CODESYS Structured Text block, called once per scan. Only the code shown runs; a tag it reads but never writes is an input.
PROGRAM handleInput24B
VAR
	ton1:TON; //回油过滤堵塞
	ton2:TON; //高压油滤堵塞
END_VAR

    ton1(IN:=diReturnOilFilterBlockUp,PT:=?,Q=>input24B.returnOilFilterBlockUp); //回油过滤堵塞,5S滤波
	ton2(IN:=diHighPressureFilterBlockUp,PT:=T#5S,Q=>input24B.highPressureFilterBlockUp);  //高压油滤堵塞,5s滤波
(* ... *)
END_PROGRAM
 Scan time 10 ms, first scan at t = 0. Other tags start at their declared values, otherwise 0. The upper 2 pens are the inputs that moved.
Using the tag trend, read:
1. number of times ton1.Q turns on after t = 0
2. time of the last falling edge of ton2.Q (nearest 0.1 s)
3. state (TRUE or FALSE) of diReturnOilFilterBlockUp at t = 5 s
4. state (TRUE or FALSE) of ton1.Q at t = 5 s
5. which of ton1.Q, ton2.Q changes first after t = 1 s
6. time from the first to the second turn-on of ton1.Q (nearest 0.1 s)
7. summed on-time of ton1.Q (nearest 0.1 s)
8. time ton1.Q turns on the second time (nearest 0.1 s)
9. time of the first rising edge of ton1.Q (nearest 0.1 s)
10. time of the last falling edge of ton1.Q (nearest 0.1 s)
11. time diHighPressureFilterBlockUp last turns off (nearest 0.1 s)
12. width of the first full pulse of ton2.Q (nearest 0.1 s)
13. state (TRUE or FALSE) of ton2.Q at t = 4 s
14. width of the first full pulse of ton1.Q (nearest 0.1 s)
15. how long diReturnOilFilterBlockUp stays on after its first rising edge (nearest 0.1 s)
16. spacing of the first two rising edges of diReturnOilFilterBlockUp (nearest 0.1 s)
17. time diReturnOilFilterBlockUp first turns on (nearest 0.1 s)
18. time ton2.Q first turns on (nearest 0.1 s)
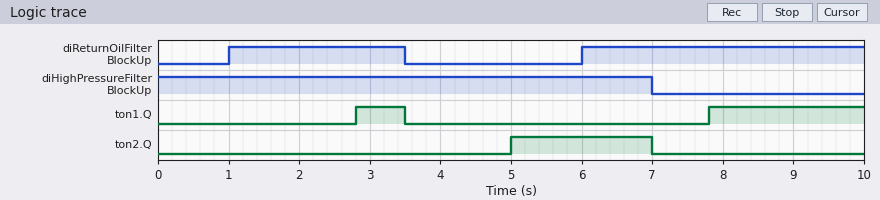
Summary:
2
7.0 s
FALSE
FALSE
ton1.Q
5.0 s
2.9 s
7.8 s
2.8 s
3.5 s
7.0 s
2.0 s
FALSE
0.7 s
2.5 s
5.0 s
1.0 s
5.0 s
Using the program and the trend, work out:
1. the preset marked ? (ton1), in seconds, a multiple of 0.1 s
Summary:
1.8 s
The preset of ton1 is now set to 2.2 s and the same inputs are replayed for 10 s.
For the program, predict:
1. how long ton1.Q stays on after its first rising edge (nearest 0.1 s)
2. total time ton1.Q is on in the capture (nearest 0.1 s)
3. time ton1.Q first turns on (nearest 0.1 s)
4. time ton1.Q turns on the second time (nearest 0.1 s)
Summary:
0.3 s
2.1 s
3.2 s
8.2 s
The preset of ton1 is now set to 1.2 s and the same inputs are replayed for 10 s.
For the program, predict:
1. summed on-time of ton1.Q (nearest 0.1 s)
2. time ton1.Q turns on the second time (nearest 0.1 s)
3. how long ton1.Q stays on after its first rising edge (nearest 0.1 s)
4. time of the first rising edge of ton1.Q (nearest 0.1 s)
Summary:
4.1 s
7.2 s
1.3 s
2.2 s
